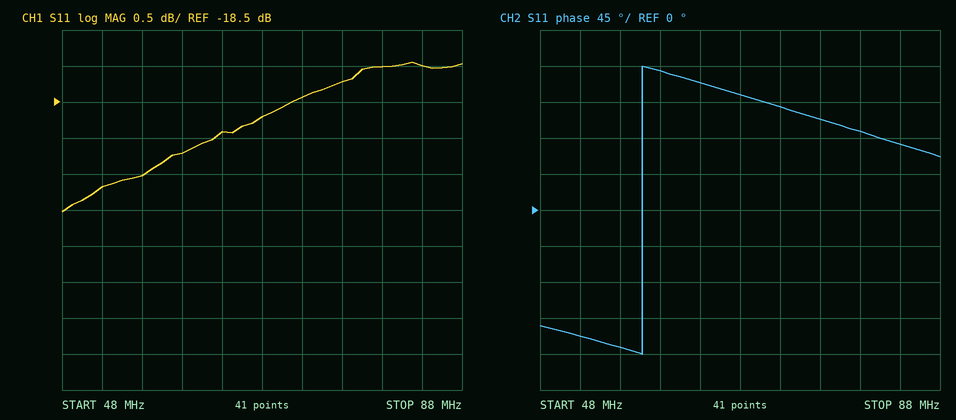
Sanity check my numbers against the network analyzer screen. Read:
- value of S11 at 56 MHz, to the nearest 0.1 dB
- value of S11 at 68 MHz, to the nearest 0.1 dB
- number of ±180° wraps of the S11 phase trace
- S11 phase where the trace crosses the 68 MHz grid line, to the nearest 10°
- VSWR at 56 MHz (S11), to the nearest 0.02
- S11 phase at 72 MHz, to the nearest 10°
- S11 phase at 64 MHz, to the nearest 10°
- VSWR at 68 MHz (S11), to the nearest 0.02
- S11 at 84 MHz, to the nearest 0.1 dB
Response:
-19.5 dB
-18.7 dB
1
140°
1.24
130°
160°
1.26
-18.0 dB
